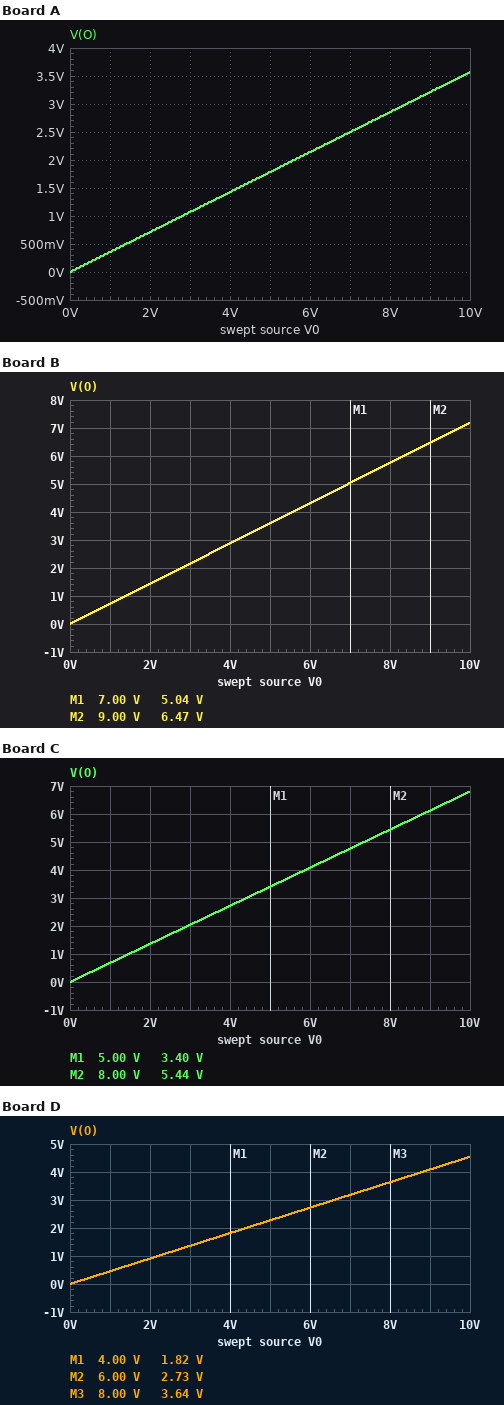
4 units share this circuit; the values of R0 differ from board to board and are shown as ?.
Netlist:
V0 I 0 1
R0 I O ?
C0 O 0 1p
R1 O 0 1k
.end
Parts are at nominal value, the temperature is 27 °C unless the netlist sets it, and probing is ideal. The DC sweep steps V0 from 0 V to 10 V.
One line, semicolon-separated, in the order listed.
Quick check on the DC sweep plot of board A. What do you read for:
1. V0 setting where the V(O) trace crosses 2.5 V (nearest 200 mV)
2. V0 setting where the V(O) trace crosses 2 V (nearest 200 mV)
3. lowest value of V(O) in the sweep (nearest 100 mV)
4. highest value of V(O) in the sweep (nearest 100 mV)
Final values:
7.0 V; 5.6 V; 0 V; 3.6 V
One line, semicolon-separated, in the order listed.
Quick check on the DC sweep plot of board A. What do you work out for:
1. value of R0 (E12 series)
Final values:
1.8 kΩ
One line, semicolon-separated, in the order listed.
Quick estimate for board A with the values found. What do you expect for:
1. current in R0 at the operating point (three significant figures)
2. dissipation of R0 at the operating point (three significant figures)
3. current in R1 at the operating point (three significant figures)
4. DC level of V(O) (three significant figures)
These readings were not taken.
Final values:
357 µA; 230 µW; 357 µA; 357 mV
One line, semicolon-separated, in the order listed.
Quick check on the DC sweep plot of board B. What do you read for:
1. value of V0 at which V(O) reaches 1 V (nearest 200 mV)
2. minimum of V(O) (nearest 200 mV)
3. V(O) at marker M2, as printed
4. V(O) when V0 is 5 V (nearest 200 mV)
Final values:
1.4 V; 0 V; 6.47 V; 3.6 V
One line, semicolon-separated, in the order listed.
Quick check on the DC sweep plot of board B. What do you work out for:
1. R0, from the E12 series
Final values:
390 Ω
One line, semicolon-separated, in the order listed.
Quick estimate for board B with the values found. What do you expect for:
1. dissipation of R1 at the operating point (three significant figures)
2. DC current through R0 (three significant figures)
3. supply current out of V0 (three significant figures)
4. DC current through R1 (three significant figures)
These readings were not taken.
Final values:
518 µW; 719 µA; 719 µA; 719 µA
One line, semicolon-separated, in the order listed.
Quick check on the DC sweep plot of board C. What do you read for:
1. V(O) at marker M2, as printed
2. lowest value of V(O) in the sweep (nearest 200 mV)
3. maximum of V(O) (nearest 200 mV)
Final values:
5.44 V; 0 V; 6.8 V
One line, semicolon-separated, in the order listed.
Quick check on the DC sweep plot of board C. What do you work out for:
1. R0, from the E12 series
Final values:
470 Ω
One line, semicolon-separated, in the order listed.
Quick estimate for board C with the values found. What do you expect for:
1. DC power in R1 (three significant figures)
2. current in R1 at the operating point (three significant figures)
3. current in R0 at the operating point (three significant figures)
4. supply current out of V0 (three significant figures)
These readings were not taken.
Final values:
463 µW; 680 µA; 680 µA; 680 µA
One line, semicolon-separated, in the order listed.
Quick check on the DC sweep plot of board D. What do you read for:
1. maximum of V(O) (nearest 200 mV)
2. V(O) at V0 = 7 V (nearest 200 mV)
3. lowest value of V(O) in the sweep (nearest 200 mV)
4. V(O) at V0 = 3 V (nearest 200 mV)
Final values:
4.6 V; 3.2 V; 0 V; 1.4 V
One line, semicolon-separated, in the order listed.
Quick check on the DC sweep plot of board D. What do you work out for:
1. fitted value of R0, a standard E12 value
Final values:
1.2 kΩ
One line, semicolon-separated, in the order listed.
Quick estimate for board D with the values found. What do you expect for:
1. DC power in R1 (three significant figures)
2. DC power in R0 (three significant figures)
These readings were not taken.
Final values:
207 µW; 248 µW
